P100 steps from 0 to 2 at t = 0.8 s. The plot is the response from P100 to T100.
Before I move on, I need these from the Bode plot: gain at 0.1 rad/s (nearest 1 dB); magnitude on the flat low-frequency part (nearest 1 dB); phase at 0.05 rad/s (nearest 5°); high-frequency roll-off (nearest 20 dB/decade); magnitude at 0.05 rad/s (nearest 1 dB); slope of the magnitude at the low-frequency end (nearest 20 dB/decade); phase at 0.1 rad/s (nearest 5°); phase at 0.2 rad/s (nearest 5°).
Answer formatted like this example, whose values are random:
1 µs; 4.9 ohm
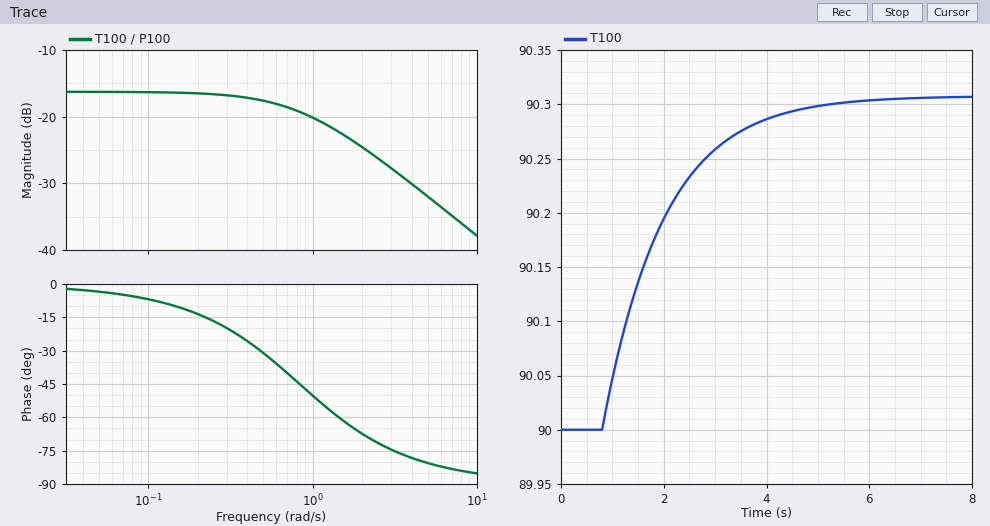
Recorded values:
-16 dB; -16 dB; -5°; -20 dB/decade; -16 dB; 0 dB/decade; -5°; -15°
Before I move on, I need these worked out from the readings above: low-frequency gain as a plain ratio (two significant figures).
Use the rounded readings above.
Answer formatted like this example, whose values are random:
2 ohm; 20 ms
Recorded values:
0.16
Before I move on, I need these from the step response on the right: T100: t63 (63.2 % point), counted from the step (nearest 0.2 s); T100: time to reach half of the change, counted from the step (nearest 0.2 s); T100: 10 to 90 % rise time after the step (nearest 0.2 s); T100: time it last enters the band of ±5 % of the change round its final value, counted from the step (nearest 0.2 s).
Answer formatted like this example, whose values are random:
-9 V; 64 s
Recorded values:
1.2 s; 0.8 s; 2.6 s; 3.6 s
